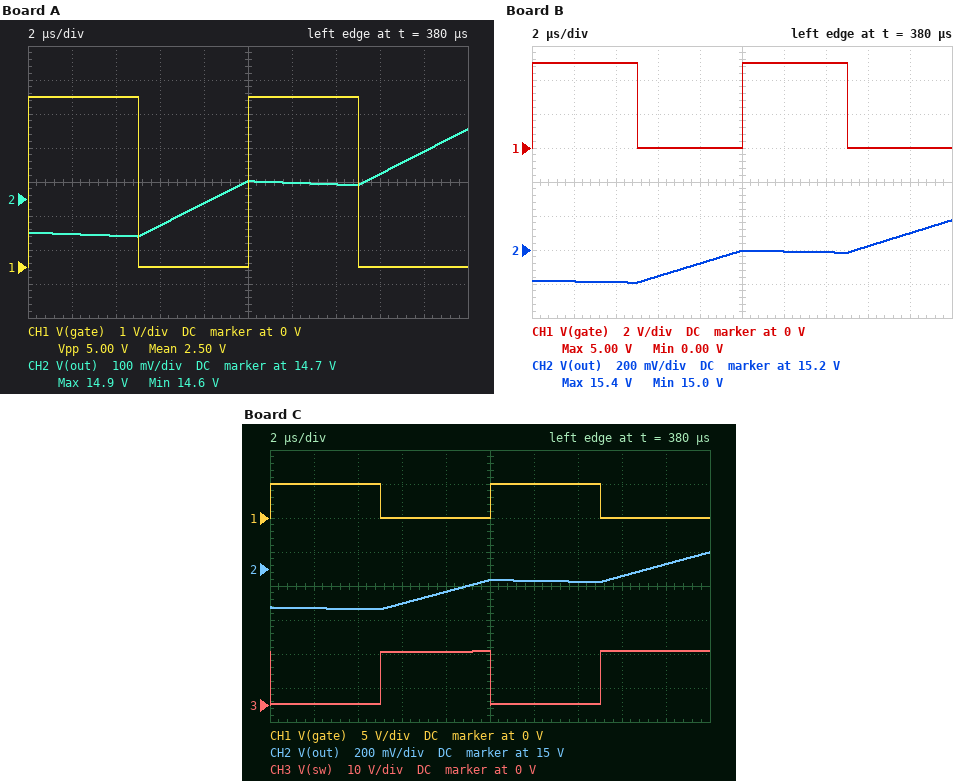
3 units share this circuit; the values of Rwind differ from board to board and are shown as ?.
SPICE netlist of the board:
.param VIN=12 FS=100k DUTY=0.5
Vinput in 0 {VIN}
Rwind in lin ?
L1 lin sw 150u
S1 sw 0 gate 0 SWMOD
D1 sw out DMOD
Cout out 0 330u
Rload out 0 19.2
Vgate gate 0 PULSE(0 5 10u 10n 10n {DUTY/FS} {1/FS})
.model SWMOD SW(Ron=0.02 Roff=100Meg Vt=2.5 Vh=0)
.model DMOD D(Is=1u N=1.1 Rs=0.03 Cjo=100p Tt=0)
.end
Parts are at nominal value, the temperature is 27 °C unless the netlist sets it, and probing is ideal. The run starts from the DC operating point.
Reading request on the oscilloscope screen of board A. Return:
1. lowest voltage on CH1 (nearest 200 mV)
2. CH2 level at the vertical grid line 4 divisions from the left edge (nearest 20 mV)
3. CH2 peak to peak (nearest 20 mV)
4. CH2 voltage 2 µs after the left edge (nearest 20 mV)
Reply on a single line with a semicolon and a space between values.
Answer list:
0 V; 14.68 V; 320 mV; 14.60 V
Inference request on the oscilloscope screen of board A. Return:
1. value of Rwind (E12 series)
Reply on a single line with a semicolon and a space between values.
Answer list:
0.15 Ω
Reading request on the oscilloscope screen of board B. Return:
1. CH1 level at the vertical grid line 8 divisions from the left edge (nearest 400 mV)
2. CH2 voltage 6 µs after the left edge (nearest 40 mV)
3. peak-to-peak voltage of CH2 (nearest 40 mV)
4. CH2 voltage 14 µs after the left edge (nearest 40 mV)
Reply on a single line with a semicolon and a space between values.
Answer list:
0 V; 15.04 V; 360 mV; 15.20 V
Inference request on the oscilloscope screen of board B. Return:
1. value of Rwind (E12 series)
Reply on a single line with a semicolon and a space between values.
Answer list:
0.033 Ω
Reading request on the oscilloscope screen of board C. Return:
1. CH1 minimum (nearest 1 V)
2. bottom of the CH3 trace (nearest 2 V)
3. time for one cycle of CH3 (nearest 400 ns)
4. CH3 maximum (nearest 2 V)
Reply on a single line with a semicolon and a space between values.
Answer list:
0 V; 0 V; 10.0 µs; 16 V
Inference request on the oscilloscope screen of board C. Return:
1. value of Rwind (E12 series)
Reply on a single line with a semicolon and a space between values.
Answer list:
0.1 Ω
